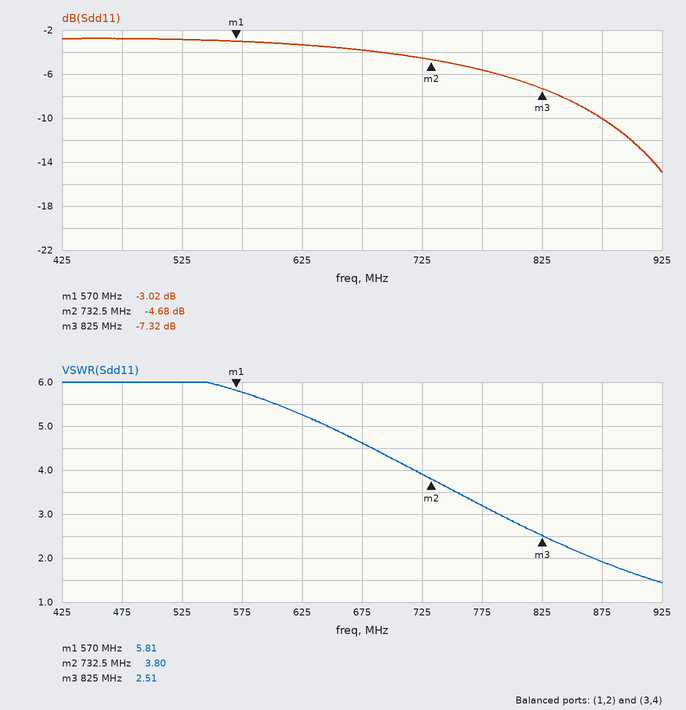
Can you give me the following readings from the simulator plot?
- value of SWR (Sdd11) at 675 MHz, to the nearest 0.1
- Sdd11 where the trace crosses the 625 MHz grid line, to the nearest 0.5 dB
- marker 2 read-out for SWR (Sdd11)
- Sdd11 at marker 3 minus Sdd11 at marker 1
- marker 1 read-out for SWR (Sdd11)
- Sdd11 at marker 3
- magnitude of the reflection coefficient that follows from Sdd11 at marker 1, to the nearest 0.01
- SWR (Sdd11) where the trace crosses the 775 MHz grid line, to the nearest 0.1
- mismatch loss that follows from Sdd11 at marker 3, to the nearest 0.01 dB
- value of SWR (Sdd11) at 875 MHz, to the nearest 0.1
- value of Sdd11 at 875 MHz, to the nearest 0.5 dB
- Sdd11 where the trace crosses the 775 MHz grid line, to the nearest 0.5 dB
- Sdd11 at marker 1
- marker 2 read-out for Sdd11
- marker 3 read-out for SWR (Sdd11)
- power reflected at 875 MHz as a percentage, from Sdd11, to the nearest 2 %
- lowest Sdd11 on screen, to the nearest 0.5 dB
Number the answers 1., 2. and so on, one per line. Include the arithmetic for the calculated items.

1. 4.6
2. -3.5 dB
3. 3.80
4. -7.32 − (-3.02) = -4.30 dB
5. 5.81
6. -7.32 dB
7. 10^(-3.02/20) ≈ 0.71
8. 3.2
9. −10 log10(1 − 10^(-7.32/10)) ≈ 0.89 dB
10. 1.9
11. -10.0 dB
12. -5.5 dB
13. -3.02 dB
14. -4.68 dB
15. 2.51
16. 10^(-10/10) ≈ 10 %
17. -15.0 dB
